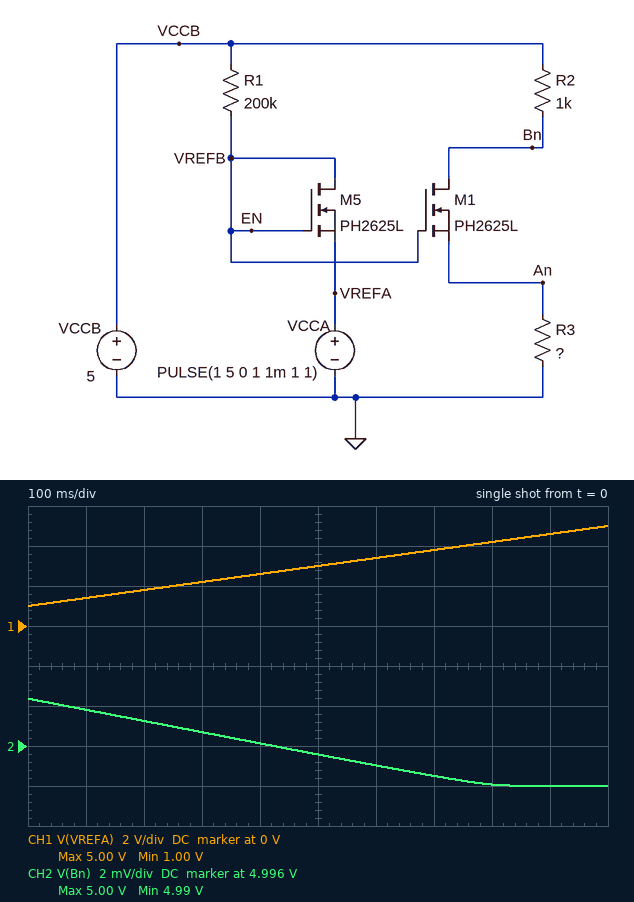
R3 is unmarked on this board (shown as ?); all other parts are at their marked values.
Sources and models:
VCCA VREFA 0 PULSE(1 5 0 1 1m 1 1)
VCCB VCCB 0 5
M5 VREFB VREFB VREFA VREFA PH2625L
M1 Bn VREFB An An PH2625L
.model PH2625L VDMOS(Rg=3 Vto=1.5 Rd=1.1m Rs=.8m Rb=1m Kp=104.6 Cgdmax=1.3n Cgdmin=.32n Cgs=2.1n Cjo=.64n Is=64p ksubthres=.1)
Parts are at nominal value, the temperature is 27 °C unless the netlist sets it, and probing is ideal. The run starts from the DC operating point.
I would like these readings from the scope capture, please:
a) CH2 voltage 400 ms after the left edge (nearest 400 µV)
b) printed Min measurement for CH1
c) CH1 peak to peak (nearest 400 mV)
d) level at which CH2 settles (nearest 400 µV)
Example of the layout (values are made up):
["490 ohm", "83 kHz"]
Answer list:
["4.9960 V", "1.00 V", "4.0 V", "4.9940 V"]
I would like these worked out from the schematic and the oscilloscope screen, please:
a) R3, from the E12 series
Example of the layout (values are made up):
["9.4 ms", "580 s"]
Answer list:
["680 kΩ"]
